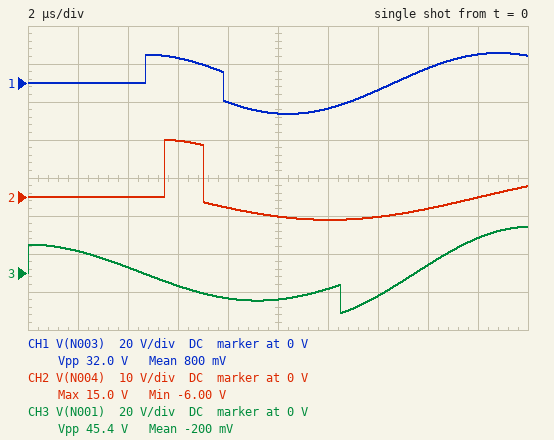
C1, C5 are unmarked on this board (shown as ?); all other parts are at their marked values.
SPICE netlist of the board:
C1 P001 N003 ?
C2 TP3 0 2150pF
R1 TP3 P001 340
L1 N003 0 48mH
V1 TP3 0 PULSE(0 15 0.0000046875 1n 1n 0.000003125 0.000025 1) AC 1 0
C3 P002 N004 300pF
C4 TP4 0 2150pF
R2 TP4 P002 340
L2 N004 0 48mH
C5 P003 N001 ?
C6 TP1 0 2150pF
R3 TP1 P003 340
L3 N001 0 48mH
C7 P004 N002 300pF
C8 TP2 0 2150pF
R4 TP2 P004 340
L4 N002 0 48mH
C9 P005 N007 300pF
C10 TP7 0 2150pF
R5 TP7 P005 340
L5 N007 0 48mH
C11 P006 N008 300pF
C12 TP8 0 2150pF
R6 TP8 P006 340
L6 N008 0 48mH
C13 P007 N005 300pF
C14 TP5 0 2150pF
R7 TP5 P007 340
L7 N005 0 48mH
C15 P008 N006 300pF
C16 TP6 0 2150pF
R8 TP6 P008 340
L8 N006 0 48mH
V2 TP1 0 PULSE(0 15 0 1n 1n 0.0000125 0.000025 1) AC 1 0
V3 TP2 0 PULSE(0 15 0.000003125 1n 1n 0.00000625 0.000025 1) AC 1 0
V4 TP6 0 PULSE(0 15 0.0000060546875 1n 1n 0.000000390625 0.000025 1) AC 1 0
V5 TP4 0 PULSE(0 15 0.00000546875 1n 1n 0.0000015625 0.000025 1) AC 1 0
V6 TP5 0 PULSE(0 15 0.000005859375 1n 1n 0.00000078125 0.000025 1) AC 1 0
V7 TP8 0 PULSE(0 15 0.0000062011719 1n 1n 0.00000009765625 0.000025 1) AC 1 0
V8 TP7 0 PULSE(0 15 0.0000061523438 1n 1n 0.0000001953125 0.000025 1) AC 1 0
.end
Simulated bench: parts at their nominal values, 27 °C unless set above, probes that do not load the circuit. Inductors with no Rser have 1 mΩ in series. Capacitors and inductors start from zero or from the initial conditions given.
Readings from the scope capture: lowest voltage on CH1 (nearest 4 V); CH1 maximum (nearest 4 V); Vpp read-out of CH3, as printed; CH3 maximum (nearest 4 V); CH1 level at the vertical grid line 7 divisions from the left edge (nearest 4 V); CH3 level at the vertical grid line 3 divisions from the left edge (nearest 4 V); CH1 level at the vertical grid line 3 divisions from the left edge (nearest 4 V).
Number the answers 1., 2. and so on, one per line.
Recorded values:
1. -16 V
2. 16 V
3. 45.4 V
4. 24 V
5. -4 V
6. -8 V
7. 12 V
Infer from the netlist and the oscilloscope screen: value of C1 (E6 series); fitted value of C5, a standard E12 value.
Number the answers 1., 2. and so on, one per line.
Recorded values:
1. 150 pF
2. 180 pF
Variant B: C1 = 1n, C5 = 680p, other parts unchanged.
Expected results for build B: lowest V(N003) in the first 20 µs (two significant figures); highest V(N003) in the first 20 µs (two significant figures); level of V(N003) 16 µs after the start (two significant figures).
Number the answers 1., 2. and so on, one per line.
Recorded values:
1. -6.5 V
2. 15 V
3. -6.4 V
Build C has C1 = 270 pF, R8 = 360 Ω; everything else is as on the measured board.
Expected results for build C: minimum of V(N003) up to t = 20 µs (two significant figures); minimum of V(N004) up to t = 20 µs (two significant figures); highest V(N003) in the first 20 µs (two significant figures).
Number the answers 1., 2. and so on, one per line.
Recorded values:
1. -12 V
2. -6.0 V
3. 15 V
